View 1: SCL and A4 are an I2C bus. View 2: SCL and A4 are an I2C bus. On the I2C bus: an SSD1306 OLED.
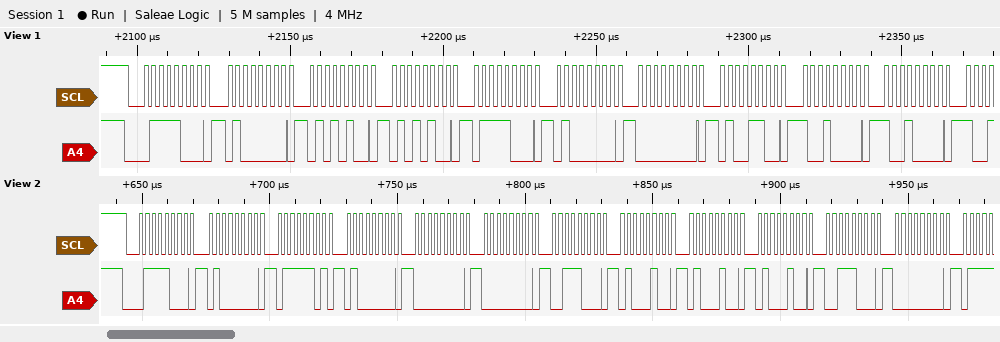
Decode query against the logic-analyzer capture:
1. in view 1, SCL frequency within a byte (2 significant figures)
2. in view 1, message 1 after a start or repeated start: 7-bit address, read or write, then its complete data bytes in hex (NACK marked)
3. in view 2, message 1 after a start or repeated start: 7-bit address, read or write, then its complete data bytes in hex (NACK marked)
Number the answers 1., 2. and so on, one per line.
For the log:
1. 400 kHz
2. 0x3C write: 40 54 54 78 40 00 4C 90 90
3. 0x3C write: 40 7D 40 00 00 38 44 44 44 38 00
